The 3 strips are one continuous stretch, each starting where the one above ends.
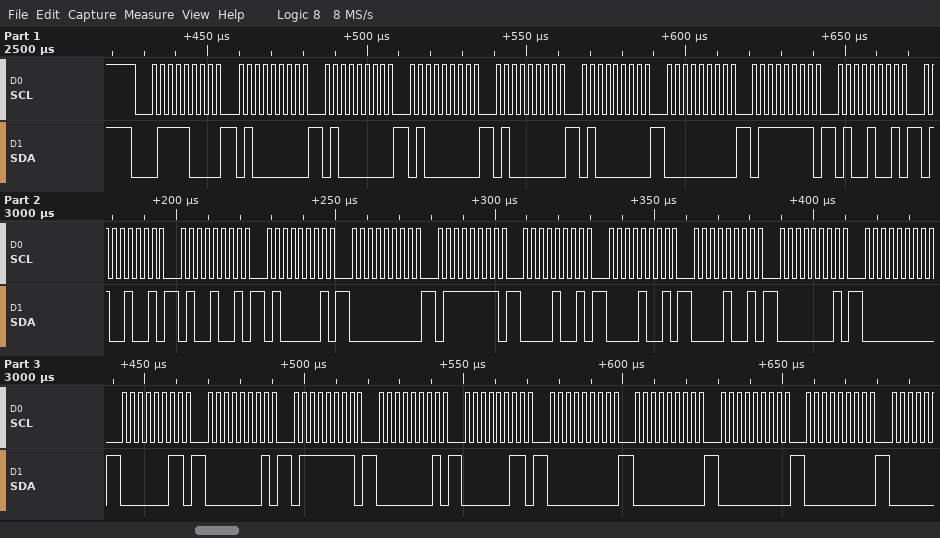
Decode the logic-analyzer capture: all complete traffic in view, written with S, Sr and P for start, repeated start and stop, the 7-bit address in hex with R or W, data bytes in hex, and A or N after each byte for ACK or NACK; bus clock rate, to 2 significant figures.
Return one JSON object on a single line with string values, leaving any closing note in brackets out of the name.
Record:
{"all complete traffic in view, written with S, Sr and P for start, repeated start and stop, the 7-bit address in hex with R or W, data bytes in hex, and A or N after each byte for ACK or NACK": "S 3CW A 40 A 40 A 40 A 40 A 40 A 00 A 7F A 49 A 49 A 49 A 41 A 00 A 7F A 09 A 09 A 09 A 01 A 00 A 03 A 01 A 7F A 01 A 03 A 00 A 00 A 00 A 00 A", "bus clock rate, to 2 significant figures": "400 kHz"}
